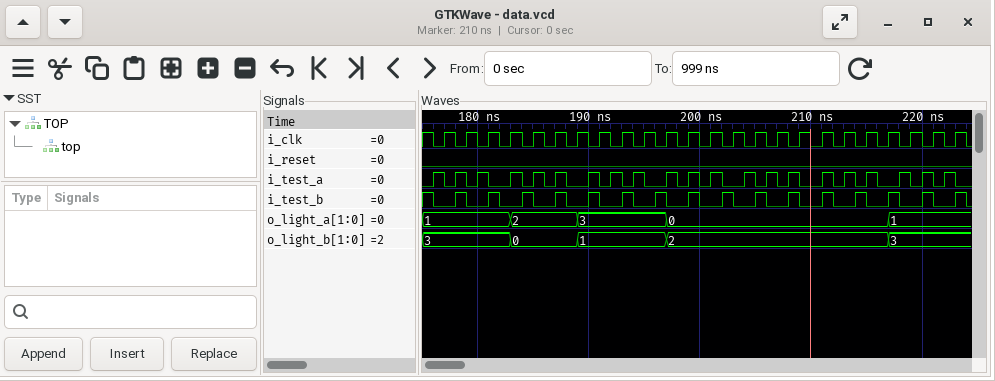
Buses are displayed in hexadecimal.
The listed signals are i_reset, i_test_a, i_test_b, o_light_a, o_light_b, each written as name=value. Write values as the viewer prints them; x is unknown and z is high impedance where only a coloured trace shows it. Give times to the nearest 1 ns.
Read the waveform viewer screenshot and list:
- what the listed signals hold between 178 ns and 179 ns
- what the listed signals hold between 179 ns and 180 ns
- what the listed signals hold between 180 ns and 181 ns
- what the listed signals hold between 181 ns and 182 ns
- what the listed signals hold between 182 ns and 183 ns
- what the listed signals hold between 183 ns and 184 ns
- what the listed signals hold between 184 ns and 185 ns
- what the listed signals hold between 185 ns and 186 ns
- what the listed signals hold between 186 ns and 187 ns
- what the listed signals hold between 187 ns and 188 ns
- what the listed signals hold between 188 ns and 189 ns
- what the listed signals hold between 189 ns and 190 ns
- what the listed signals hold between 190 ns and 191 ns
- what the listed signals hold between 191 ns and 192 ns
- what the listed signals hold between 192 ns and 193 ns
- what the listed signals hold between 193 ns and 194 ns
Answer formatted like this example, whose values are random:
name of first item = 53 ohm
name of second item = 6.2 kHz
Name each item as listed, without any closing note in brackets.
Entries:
what the listed signals hold between 178 ns and 179 ns = i_reset=0, i_test_a=1, i_test_b=1, o_light_a=1, o_light_b=3
what the listed signals hold between 179 ns and 180 ns = i_reset=0, i_test_a=0, i_test_b=0, o_light_a=1, o_light_b=3
what the listed signals hold between 180 ns and 181 ns = i_reset=0, i_test_a=1, i_test_b=0, o_light_a=1, o_light_b=3
what the listed signals hold between 181 ns and 182 ns = i_reset=0, i_test_a=0, i_test_b=1, o_light_a=1, o_light_b=3
what the listed signals hold between 182 ns and 183 ns = i_reset=0, i_test_a=0, i_test_b=0, o_light_a=1, o_light_b=3
what the listed signals hold between 183 ns and 184 ns = i_reset=0, i_test_a=1, i_test_b=0, o_light_a=2, o_light_b=0
what the listed signals hold between 184 ns and 185 ns = i_reset=0, i_test_a=0, i_test_b=1, o_light_a=2, o_light_b=0
what the listed signals hold between 185 ns and 186 ns = i_reset=0, i_test_a=1, i_test_b=0, o_light_a=2, o_light_b=0
what the listed signals hold between 186 ns and 187 ns = i_reset=0, i_test_a=0, i_test_b=0, o_light_a=2, o_light_b=0
what the listed signals hold between 187 ns and 188 ns = i_reset=0, i_test_a=1, i_test_b=1, o_light_a=2, o_light_b=0
what the listed signals hold between 188 ns and 189 ns = i_reset=0, i_test_a=0, i_test_b=0, o_light_a=2, o_light_b=0
what the listed signals hold between 189 ns and 190 ns = i_reset=0, i_test_a=0, i_test_b=0, o_light_a=3, o_light_b=1
what the listed signals hold between 190 ns and 191 ns = i_reset=0, i_test_a=1, i_test_b=1, o_light_a=3, o_light_b=1
what the listed signals hold between 191 ns and 192 ns = i_reset=0, i_test_a=0, i_test_b=0, o_light_a=3, o_light_b=1
what the listed signals hold between 192 ns and 193 ns = i_reset=0, i_test_a=1, i_test_b=0, o_light_a=3, o_light_b=1
what the listed signals hold between 193 ns and 194 ns = i_reset=0, i_test_a=0, i_test_b=1, o_light_a=3, o_light_b=1
